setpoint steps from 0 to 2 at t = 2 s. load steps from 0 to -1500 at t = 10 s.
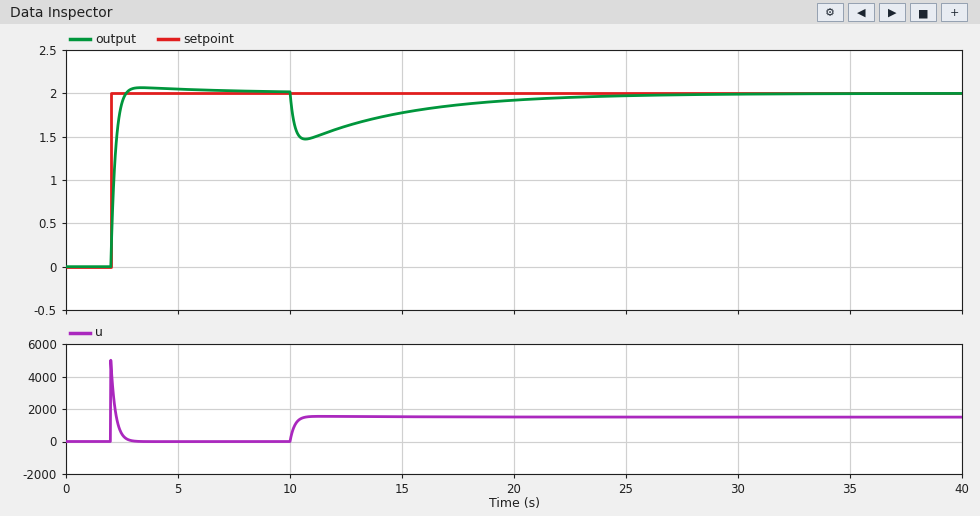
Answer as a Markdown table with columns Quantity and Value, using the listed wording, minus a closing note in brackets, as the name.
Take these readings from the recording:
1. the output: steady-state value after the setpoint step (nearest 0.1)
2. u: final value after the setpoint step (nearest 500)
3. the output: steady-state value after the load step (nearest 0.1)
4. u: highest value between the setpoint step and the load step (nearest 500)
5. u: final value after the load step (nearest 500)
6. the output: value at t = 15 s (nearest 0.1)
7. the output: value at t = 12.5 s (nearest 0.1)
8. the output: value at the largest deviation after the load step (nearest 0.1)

| Quantity | Value |
|---|---|
| the output: steady-state value after the setpoint step | 2.0 |
| u: final value after the setpoint step | 0 |
| the output: steady-state value after the load step | 2.0 |
| u: highest value between the setpoint step and the load step | 5000 |
| u: final value after the load step | 1500 |
| the output: value at t = 15 s | 1.8 |
| the output: value at t = 12.5 s | 1.6 |
| the output: value at the largest deviation after the load step | 1.5 |
